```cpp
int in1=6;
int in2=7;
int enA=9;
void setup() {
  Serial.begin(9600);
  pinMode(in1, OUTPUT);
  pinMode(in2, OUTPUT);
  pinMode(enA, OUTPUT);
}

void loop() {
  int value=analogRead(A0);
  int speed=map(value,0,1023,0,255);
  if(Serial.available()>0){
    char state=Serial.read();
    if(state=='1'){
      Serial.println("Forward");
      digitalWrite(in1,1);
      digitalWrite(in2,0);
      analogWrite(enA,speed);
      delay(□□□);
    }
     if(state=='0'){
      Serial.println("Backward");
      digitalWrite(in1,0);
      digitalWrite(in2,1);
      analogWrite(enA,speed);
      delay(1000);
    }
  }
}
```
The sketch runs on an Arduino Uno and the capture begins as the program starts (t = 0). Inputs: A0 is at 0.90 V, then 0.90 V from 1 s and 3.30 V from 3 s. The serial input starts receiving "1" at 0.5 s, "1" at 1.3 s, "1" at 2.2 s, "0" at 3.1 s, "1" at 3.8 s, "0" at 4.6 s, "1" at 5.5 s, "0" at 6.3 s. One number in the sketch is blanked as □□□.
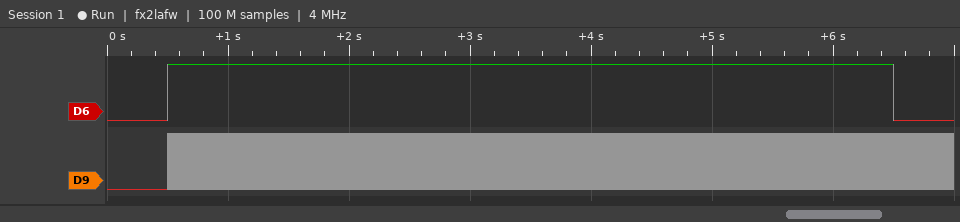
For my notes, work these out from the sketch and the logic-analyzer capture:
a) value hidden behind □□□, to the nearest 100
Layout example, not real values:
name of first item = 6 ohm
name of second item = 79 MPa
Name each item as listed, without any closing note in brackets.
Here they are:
value hidden behind □□□, to the nearest 100 = 2000
